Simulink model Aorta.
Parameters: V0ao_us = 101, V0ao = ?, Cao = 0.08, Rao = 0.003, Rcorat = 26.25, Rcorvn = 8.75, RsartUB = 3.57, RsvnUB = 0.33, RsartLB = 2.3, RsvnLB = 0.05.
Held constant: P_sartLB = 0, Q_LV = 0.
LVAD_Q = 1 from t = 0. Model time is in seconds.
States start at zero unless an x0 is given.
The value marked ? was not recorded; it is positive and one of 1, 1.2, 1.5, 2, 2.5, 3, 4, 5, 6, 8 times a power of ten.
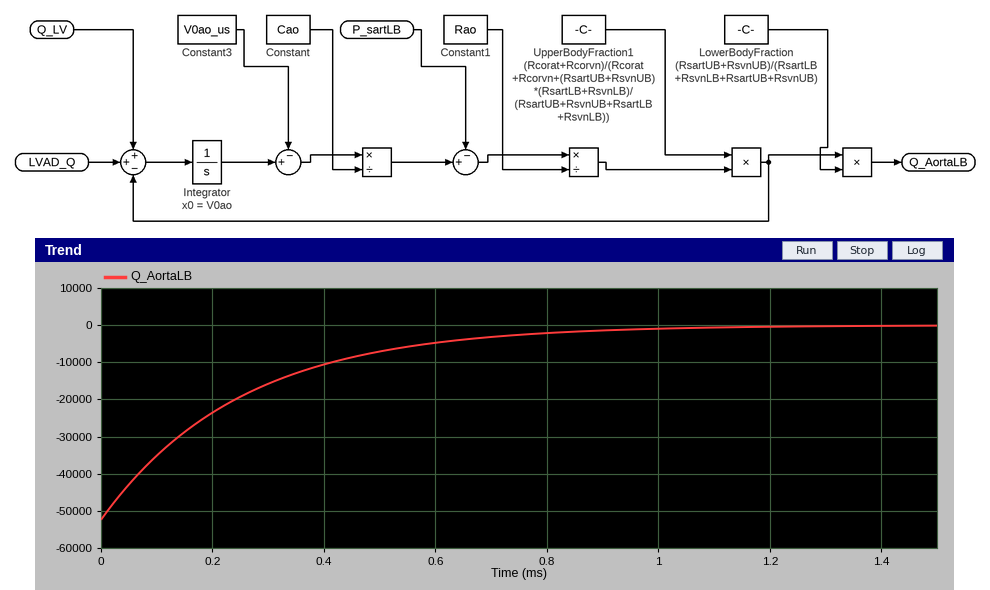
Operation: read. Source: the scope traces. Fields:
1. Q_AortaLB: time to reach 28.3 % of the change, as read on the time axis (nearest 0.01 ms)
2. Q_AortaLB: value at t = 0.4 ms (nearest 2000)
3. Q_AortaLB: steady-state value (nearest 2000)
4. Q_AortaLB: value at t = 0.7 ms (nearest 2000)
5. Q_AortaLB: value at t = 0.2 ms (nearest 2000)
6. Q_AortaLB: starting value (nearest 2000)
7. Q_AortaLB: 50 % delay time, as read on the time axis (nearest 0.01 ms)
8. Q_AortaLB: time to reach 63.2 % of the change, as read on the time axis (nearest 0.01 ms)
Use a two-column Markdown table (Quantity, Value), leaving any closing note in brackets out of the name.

| Quantity | Value |
|---|---|
| Q_AortaLB: time to reach 28.3 % of the change, as read on the time axis | 0.08 ms |
| Q_AortaLB: value at t = 0.4 ms | -10000 |
| Q_AortaLB: steady-state value | 0 |
| Q_AortaLB: value at t = 0.7 ms | -4000 |
| Q_AortaLB: value at t = 0.2 ms | -24000 |
| Q_AortaLB: starting value | -52000 |
| Q_AortaLB: 50 % delay time, as read on the time axis | 0.17 ms |
| Q_AortaLB: time to reach 63.2 % of the change, as read on the time axis | 0.25 ms |
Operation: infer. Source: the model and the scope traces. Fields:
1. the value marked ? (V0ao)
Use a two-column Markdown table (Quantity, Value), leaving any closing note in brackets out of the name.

| Quantity | Value |
|---|---|
| the value marked ? | 80 |
